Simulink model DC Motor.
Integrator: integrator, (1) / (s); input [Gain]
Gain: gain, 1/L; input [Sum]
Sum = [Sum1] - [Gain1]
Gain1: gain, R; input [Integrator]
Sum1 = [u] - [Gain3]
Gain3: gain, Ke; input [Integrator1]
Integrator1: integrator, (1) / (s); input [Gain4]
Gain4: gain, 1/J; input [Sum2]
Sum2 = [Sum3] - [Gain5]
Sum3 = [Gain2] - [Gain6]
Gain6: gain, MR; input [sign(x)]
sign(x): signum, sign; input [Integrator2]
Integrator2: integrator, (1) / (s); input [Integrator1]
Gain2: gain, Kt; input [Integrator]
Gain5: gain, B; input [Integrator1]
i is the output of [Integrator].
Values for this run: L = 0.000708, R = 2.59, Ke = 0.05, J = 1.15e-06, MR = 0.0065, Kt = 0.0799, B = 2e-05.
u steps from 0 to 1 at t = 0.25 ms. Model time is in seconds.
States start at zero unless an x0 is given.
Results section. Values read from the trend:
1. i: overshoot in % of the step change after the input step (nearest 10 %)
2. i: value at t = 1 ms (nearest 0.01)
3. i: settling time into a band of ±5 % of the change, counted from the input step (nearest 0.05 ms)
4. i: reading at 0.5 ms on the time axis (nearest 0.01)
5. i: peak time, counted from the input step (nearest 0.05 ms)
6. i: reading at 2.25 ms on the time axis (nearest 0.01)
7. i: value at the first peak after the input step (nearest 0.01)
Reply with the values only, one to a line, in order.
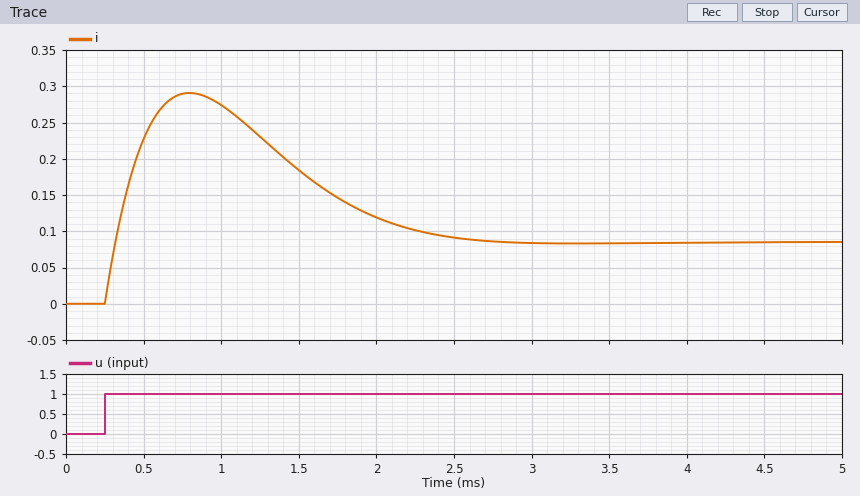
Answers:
240 %
0.27
2.30 ms
0.23
0.55 ms
0.10
0.29
